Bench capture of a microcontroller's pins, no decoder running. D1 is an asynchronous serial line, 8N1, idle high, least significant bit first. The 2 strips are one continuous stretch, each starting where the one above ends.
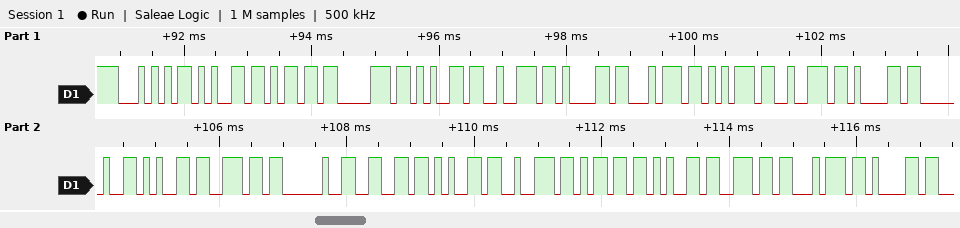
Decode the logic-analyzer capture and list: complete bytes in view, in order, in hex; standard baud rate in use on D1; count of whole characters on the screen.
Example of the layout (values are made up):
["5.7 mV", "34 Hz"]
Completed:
["54 65 6D 70 65 72 61 74 75 72 61 20 65 6E 20 66 65 72 6D 65 6E 74 61", "9600 baud", "23"]
